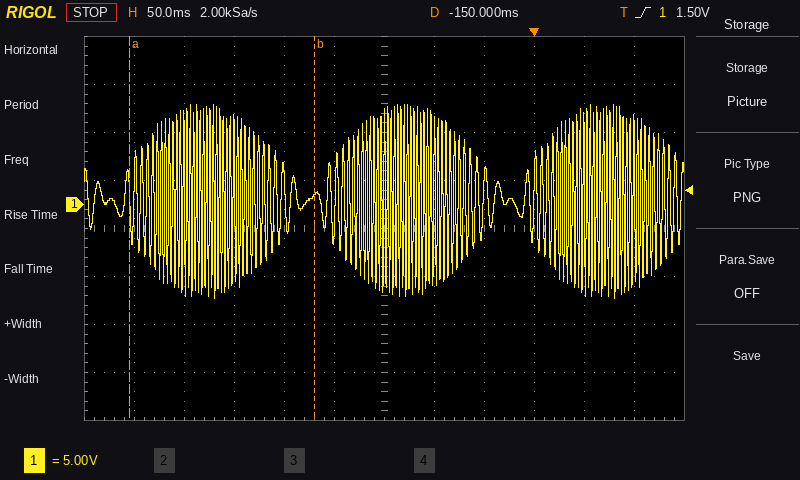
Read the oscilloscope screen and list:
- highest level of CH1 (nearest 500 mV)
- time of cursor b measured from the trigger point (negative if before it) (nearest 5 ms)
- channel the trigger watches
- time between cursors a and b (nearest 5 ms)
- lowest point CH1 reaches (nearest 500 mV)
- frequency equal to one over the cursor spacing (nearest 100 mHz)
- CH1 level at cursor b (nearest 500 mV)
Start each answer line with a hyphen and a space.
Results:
- 10.5 V
- -220 ms
- CH1
- 185 ms
- -10.0 V
- 5.4 Hz
- 1.0 V
